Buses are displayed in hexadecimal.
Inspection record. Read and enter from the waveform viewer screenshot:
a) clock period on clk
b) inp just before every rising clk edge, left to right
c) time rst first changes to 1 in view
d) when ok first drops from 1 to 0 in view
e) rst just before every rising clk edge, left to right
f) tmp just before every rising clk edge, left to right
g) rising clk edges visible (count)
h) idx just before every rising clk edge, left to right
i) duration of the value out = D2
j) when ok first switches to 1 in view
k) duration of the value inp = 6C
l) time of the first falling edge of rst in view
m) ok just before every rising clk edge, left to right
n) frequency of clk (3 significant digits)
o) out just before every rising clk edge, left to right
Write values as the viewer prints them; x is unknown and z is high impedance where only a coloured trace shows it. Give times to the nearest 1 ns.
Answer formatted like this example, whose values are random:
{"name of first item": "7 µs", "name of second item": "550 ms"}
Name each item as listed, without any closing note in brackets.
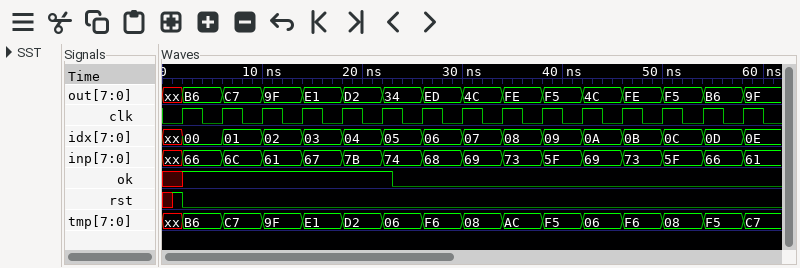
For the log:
{"clock period on clk": "4 ns", "inp just before every rising clk edge, left to right": "xx, 66, 6C, 61, 67, 7B, 74, 68, 69, 73, 5F, 69, 73, 5F, 66", "time rst first changes to 1 in view": "1 ns", "when ok first drops from 1 to 0 in view": "23 ns", "rst just before every rising clk edge, left to right": "1 0 0 0 0 0 0 0 0 0 0 0 0 0 0", "tmp just before every rising clk edge, left to right": "xx, B6, C7, 9F, E1, D2, 06, F6, 08, AC, F5, 06, F6, 08, F5", "rising clk edges visible": "15", "idx just before every rising clk edge, left to right": "xx, 00, 01, 02, 03, 04, 05, 06, 07, 08, 09, 0A, 0B, 0C, 0D", "duration of the value out = D2": "4 ns", "when ok first switches to 1 in view": "2 ns", "duration of the value inp = 6C": "4 ns", "time of the first falling edge of rst in view": "2 ns", "ok just before every rising clk edge, left to right": "x 1 1 1 1 1 0 0 0 0 0 0 0 0 0", "frequency of clk": "250 MHz", "out just before every rising clk edge, left to right": "xx, B6, C7, 9F, E1, D2, 34, ED, 4C, FE, F5, 4C, FE, F5, B6"}
